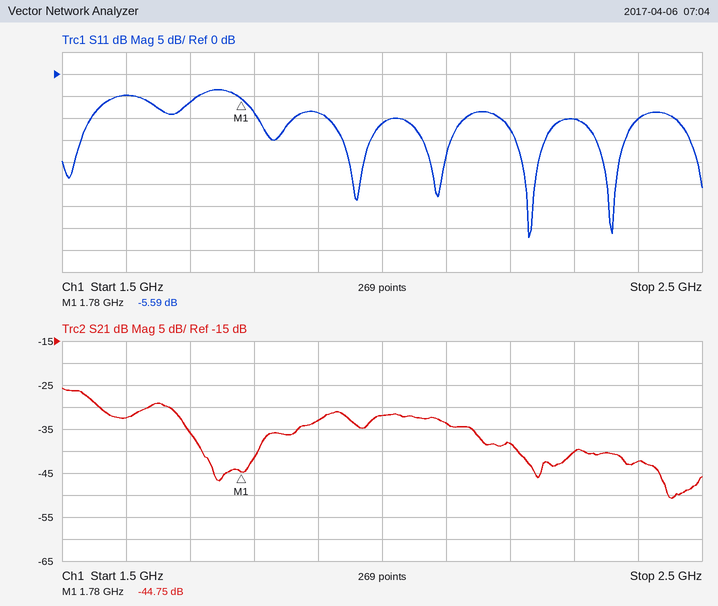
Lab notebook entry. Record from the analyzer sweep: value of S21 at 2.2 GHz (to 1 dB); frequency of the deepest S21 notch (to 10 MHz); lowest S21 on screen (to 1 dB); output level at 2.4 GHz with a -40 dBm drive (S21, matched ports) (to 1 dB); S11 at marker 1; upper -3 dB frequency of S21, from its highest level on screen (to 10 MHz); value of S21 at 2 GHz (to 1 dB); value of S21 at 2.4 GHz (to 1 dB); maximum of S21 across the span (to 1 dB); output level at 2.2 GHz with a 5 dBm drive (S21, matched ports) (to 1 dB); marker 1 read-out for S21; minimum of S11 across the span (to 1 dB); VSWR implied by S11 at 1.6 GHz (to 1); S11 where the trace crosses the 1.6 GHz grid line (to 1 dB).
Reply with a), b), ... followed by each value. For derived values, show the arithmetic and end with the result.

a) -38 dB
b) 2.45 GHz
c) -51 dB
d) -40 dBm + (-42 dB) = -82 dBm
e) -5.59 dB
f) 1.55 GHz
g) -32 dB
h) -42 dB
i) -26 dB
j) 5 dBm + (-38 dB) = -33 dBm
k) -44.75 dB
l) -37 dB
m) |Γ| = 10^(-5/20) = 0.5623; VSWR = (1 + 0.5623)/(1 − 0.5623) ≈ 4
n) -5 dB
